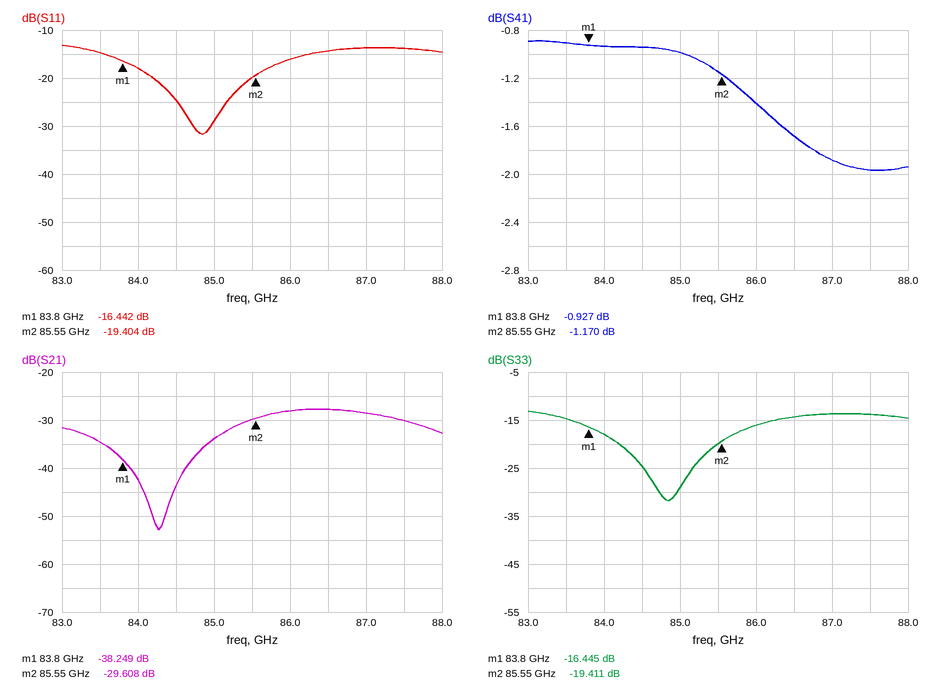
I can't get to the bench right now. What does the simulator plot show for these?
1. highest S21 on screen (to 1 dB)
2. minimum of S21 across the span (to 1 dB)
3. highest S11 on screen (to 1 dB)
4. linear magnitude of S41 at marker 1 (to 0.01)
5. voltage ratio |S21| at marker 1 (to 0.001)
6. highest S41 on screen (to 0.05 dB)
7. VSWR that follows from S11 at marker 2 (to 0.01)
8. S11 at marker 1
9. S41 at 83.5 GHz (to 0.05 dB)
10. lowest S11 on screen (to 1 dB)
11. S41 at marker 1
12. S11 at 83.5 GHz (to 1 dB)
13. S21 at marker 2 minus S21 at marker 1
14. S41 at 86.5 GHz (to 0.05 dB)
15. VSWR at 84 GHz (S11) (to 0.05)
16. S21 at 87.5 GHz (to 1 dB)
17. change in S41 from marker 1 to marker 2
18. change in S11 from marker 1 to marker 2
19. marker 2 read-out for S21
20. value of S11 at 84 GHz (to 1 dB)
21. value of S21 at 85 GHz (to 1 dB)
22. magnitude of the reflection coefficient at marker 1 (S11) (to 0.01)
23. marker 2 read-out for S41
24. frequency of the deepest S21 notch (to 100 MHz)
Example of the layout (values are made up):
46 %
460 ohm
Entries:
-28 dB
-53 dB
-13 dB
0.90
0.012
-0.90 dB
1.24
-16.442 dB
-0.90 dB
-32 dB
-0.927 dB
-15 dB
8.641 dB
-1.70 dB
1.30
-30 dB
-0.243 dB
-2.962 dB
-29.608 dB
-18 dB
-34 dB
0.15
-1.170 dB
84.3 GHz
